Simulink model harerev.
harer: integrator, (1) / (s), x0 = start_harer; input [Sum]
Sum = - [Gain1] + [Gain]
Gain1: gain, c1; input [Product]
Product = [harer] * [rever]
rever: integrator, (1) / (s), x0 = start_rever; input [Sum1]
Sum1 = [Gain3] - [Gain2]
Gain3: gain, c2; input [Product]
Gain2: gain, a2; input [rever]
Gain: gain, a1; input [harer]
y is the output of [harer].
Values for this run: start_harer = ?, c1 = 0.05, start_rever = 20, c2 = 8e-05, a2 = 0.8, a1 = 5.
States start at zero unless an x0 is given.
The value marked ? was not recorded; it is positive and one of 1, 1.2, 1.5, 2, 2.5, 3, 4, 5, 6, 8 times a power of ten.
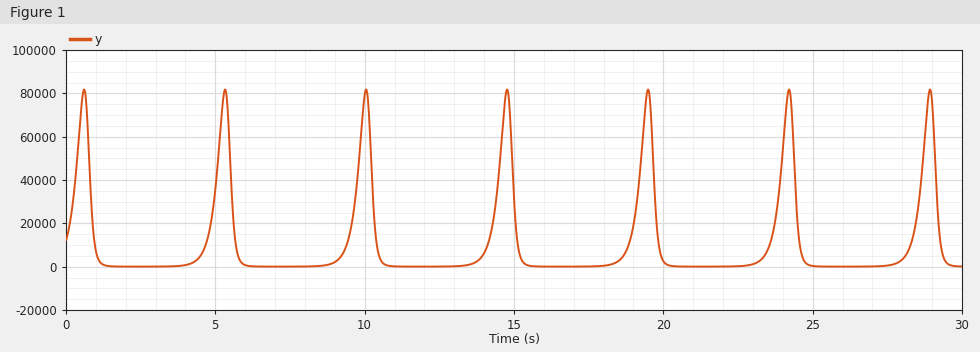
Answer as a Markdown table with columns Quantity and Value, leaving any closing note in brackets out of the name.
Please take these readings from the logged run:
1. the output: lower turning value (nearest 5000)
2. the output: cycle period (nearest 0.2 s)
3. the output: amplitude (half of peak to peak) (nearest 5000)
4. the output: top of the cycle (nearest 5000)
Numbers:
| Quantity | Value |
|---|---|
| the output: lower turning value | 0 |
| the output: cycle period | 4.8 s |
| the output: amplitude (half of peak to peak) | 40000 |
| the output: top of the cycle | 80000 |
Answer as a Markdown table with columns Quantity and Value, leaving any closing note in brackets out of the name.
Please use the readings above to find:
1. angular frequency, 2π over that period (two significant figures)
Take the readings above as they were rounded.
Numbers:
| Quantity | Value |
|---|---|
| angular frequency, 2π over that period | 1.3 rad/s |
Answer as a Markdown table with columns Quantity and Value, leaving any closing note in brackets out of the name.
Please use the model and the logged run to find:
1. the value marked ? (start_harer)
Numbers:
| Quantity | Value |
|---|---|
| the value marked ? | 12000 |
